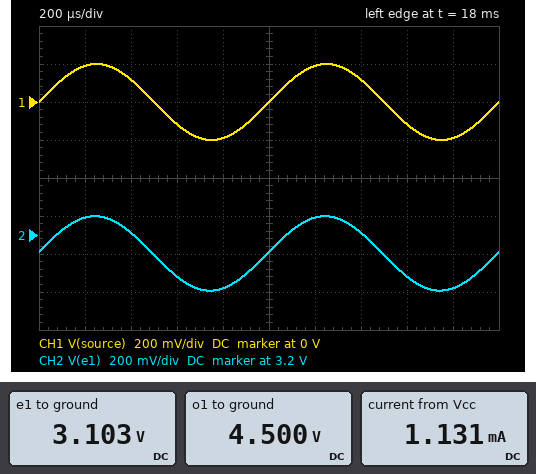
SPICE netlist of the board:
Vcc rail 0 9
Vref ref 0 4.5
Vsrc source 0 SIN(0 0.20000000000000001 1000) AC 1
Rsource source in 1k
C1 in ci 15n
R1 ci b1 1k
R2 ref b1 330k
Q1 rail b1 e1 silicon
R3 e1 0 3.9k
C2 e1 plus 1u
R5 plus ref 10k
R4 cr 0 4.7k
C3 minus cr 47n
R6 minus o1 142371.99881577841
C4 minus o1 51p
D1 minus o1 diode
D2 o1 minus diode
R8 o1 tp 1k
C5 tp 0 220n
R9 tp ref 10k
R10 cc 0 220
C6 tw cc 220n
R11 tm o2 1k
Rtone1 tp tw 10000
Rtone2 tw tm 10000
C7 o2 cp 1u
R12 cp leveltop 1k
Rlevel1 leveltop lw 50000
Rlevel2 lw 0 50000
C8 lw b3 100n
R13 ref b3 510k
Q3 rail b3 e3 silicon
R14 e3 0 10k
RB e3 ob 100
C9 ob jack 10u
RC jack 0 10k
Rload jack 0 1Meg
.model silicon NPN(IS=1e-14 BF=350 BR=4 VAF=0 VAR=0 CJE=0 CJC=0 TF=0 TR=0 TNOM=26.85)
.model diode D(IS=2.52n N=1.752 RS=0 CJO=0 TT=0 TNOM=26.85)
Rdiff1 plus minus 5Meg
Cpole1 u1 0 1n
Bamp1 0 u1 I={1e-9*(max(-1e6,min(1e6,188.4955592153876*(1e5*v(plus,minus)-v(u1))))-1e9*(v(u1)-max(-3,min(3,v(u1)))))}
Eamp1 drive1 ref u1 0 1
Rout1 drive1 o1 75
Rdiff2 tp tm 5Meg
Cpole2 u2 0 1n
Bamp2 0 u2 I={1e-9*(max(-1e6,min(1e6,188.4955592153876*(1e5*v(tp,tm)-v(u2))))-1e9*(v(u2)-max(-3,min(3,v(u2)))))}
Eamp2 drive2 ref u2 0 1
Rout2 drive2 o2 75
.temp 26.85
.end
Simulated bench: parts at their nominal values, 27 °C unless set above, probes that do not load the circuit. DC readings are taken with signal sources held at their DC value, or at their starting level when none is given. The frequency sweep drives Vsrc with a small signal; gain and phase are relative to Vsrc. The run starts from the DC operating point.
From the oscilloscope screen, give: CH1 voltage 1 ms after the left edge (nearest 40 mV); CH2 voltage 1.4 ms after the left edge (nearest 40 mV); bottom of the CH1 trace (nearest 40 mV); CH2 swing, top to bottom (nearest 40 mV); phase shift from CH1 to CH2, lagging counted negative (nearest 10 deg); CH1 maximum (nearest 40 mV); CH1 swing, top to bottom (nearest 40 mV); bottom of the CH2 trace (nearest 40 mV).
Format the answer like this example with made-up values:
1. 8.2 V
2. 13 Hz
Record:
1. 0 V
2. 3.20 V
3. -200 mV
4. 400 mV
5. 0 deg
6. 200 mV
7. 400 mV
8. 2.92 V
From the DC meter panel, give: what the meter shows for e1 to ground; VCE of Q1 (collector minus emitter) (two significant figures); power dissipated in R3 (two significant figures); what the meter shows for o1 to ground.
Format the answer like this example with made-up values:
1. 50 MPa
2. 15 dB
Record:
1. 3.103 V
2. 5.9 V
3. 2.5 mW
4. 4.500 V
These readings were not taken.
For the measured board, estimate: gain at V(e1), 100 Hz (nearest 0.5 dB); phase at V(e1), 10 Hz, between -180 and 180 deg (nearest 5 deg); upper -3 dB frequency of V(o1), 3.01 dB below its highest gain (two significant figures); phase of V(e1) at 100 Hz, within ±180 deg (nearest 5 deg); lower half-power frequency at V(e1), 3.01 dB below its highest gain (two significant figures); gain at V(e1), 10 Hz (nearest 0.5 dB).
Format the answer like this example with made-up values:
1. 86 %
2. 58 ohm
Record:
1. -1.0 dB
2. 75 deg
3. 19 kHz
4. 25 deg
5. 43 Hz
6. -12.5 dB
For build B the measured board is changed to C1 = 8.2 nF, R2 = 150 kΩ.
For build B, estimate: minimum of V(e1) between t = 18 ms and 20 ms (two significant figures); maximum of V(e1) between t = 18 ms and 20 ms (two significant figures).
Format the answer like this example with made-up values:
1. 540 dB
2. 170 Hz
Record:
1. 3.3 V
2. 3.7 V
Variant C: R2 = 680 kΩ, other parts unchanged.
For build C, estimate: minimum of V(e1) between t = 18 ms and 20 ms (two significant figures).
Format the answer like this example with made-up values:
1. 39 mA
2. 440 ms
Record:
1. 2.4 V
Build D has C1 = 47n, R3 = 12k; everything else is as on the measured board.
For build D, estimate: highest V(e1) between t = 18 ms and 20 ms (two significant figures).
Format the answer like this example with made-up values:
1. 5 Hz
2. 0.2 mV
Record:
1. 3.8 V
